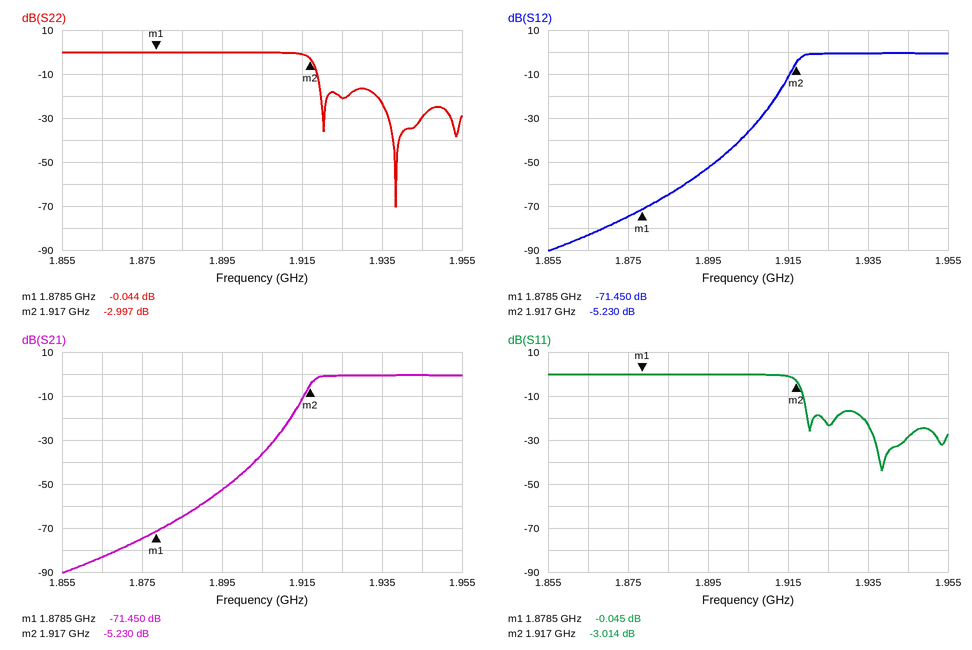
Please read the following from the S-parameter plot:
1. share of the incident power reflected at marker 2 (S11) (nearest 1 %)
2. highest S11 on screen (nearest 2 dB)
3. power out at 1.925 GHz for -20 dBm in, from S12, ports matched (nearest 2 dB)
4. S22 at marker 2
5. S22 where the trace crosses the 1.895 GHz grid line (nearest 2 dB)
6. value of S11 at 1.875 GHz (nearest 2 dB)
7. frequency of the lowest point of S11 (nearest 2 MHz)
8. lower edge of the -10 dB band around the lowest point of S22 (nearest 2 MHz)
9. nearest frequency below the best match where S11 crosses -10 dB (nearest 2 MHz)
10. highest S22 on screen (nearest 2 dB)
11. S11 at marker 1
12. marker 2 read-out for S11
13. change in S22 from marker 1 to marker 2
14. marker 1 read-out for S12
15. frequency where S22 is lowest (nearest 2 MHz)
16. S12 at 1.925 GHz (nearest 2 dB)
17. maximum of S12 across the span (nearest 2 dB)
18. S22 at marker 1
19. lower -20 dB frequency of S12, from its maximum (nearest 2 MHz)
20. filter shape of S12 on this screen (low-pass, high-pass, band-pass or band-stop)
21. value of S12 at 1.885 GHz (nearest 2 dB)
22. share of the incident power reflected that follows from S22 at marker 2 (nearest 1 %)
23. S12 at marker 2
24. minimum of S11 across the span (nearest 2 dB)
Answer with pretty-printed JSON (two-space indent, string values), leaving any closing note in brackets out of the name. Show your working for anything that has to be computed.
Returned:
{
  "share of the incident power reflected at marker 2 (S11)": "10^(-3.014/10) ≈ 50 %",
  "highest S11 on screen": "0 dB",
  "power out at 1.925 GHz for -20 dBm in, from S12, ports matched": "-20 dBm + (0 dB) = -20 dBm",
  "S22 at marker 2": "-2.997 dB",
  "S22 where the trace crosses the 1.895 GHz grid line": "0 dB",
  "value of S11 at 1.875 GHz": "0 dB",
  "frequency of the lowest point of S11": "1.938 GHz",
  "lower edge of the -10 dB band around the lowest point of S22": "1.918 GHz",
  "nearest frequency below the best match where S11 crosses -10 dB": "1.918 GHz",
  "highest S22 on screen": "0 dB",
  "S11 at marker 1": "-0.045 dB",
  "marker 2 read-out for S11": "-3.014 dB",
  "change in S22 from marker 1 to marker 2": "-2.997 − (-0.044) = -2.953 dB",
  "marker 1 read-out for S12": "-71.450 dB",
  "frequency where S22 is lowest": "1.938 GHz",
  "S12 at 1.925 GHz": "0 dB",
  "maximum of S12 across the span": "0 dB",
  "S22 at marker 1": "-0.044 dB",
  "lower -20 dB frequency of S12, from its maximum": "1.912 GHz",
  "filter shape of S12 on this screen": "high-pass",
  "value of S12 at 1.885 GHz": "-64 dB",
  "share of the incident power reflected that follows from S22 at marker 2": "10^(-2.997/10) ≈ 50 %",
  "S12 at marker 2": "-5.230 dB",
  "minimum of S11 across the span": "-44 dB"
}
